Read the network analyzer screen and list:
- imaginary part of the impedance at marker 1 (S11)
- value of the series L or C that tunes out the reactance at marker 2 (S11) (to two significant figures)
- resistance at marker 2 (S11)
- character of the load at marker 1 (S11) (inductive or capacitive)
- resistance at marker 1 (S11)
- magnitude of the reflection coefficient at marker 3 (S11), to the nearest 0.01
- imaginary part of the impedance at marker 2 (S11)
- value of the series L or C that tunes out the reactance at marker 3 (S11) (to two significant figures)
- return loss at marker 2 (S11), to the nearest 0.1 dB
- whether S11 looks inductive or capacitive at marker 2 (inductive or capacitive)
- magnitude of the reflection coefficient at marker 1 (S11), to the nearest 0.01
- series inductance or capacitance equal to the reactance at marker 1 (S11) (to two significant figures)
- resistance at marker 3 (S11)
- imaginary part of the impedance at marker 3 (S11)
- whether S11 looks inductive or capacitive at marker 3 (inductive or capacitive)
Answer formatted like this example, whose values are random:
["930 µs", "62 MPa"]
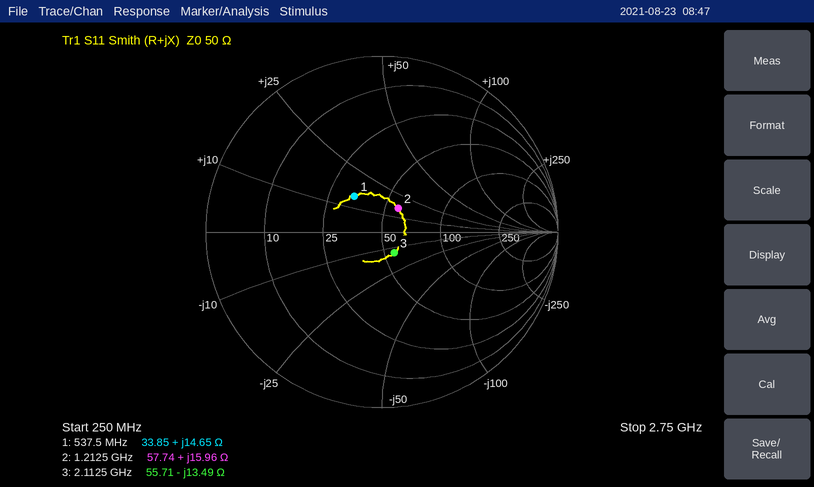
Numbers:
["+14.65 Ω", "8.2 pF", "57.74 Ω", "inductive", "33.85 Ω", "0.14", "+15.96 Ω", "1.0 nH", "15.8 dB", "inductive", "0.26", "4.3 nH", "55.71 Ω", "-13.49 Ω", "capacitive"]
